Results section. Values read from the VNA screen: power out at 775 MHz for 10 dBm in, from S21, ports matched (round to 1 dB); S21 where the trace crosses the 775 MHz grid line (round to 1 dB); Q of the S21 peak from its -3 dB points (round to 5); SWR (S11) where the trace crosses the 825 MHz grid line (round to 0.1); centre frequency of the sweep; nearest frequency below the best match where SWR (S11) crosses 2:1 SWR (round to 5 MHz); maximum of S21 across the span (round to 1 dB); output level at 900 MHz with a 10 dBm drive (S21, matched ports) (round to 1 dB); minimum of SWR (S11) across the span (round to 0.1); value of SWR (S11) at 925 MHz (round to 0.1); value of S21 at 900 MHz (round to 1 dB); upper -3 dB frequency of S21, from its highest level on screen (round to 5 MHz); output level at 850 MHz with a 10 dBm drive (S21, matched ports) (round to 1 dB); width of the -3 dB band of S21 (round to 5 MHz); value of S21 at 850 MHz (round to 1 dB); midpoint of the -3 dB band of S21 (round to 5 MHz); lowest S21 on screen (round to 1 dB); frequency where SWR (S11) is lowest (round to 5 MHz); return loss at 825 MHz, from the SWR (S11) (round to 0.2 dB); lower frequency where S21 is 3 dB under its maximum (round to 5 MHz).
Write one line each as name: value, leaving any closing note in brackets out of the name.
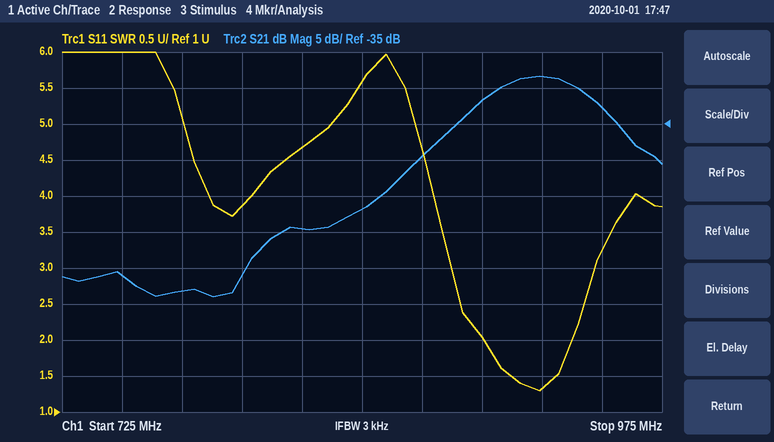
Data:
power out at 775 MHz for 10 dBm in, from S21, ports matched: -48 dBm
S21 where the trace crosses the 775 MHz grid line: -58 dB
Q of the S21 peak from its -3 dB points: 20
SWR (S11) where the trace crosses the 825 MHz grid line: 4.7
centre frequency of the sweep: 850 MHz
nearest frequency below the best match where SWR (S11) crosses 2:1 SWR: 900 MHz
maximum of S21 across the span: -28 dB
output level at 900 MHz with a 10 dBm drive (S21, matched ports): -22 dBm
minimum of SWR (S11) across the span: 1.3
value of SWR (S11) at 925 MHz: 1.3
value of S21 at 900 MHz: -32 dB
upper -3 dB frequency of S21, from its highest level on screen: 945 MHz
output level at 850 MHz with a 10 dBm drive (S21, matched ports): -37 dBm
width of the -3 dB band of S21: 45 MHz
value of S21 at 850 MHz: -47 dB
midpoint of the -3 dB band of S21: 925 MHz
lowest S21 on screen: -59 dB
frequency where SWR (S11) is lowest: 925 MHz
return loss at 825 MHz, from the SWR (S11): 3.8 dB
lower frequency where S21 is 3 dB under its maximum: 900 MHz
